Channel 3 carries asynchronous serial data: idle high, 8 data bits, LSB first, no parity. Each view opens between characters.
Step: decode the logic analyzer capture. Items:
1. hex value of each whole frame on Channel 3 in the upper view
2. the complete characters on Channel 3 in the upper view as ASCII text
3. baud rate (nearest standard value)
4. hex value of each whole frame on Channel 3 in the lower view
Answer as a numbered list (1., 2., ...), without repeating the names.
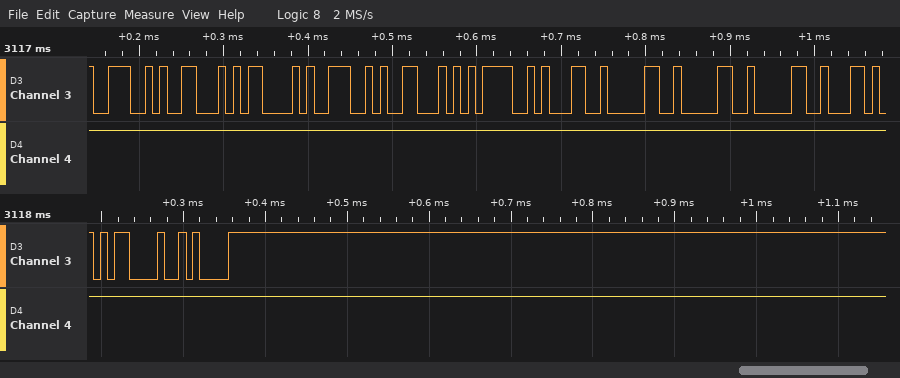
1. 4E, 46, 43, 4E, 46, 3D, 31, 30, 30, 30
2. "NFCNF=1000"
3. 115200 baud
4. 0D, 0A
